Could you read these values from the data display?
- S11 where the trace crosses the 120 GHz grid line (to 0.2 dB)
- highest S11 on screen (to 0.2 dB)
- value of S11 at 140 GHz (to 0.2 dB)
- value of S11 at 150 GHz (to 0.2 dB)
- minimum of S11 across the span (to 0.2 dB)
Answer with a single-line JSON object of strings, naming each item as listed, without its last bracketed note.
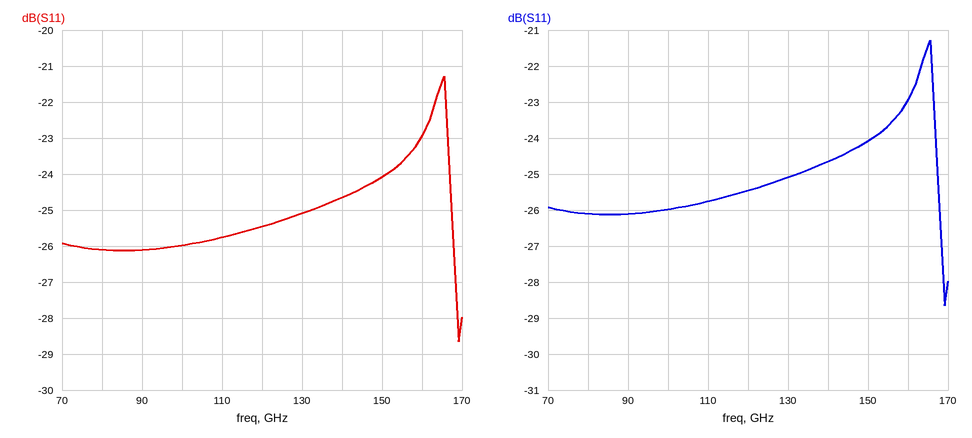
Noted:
{"S11 where the trace crosses the 120 GHz grid line": "-25.4 dB", "highest S11 on screen": "-21.2 dB", "value of S11 at 140 GHz": "-24.6 dB", "value of S11 at 150 GHz": "-24.0 dB", "minimum of S11 across the span": "-28.6 dB"}
